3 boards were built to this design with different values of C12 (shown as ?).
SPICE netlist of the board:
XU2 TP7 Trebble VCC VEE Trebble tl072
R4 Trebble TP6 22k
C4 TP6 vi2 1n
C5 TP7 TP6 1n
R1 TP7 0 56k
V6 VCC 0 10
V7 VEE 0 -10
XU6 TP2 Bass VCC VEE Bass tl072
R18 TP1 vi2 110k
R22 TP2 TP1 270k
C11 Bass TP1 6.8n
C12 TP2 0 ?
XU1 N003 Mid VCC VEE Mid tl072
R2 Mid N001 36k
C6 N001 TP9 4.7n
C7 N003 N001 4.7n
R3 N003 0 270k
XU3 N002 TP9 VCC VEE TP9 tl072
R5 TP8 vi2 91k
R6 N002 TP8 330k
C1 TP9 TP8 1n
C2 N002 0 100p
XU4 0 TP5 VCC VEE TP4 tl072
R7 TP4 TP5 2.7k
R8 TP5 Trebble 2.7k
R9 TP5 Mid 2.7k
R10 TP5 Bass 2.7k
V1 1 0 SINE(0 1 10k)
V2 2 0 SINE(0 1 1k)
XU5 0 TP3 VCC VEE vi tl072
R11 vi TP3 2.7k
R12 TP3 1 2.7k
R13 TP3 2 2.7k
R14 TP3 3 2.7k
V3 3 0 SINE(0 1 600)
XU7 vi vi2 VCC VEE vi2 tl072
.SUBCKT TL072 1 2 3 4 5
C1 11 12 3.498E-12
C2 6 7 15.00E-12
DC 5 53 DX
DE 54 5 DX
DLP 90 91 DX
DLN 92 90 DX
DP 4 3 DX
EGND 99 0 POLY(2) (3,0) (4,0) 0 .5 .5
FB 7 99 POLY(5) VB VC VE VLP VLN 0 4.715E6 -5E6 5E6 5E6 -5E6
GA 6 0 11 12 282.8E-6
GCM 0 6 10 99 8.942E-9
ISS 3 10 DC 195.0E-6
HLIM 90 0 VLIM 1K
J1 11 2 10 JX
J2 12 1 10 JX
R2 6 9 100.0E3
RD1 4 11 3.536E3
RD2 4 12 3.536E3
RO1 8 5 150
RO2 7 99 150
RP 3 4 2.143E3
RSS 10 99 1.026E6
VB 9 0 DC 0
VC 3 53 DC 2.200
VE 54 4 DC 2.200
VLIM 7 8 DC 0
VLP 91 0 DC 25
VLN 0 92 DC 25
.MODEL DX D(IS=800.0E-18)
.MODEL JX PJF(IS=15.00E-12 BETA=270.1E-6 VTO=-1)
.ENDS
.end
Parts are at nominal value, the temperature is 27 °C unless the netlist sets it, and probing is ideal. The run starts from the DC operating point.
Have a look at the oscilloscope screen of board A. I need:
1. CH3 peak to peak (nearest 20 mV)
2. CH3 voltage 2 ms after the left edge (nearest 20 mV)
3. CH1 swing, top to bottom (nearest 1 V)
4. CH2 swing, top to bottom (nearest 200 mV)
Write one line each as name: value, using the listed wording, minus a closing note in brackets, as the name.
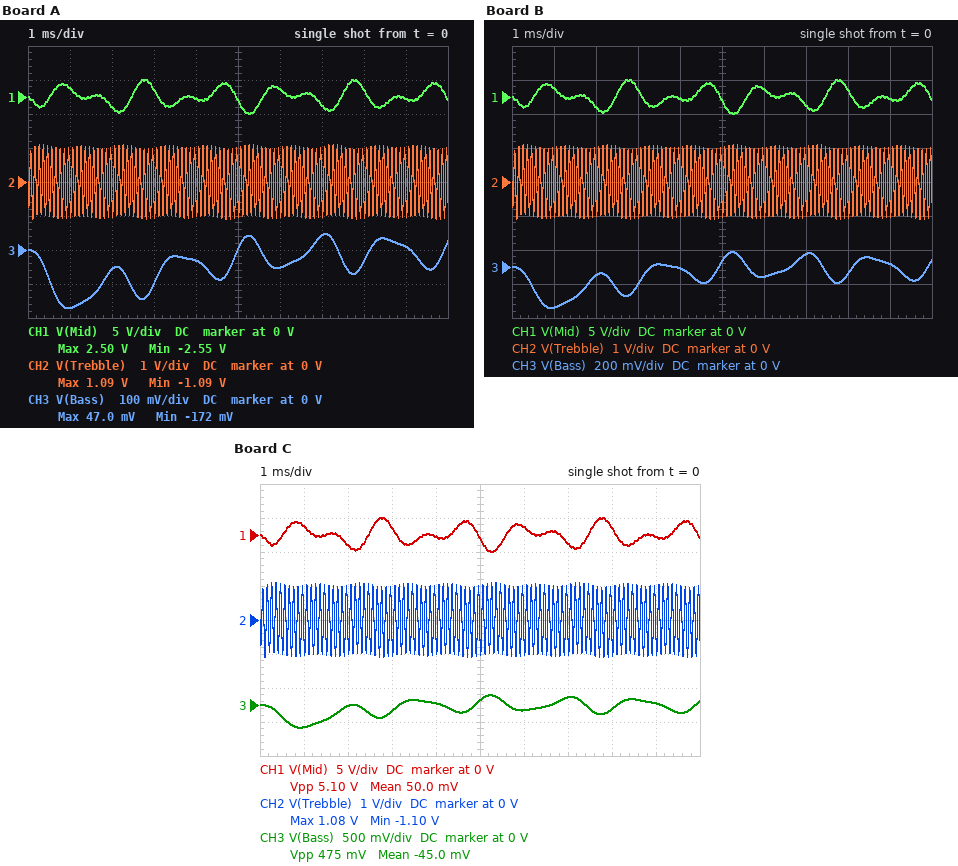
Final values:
CH3 peak to peak: 220 mV
CH3 voltage 2 ms after the left edge: -60 mV
CH1 swing, top to bottom: 5 V
CH2 swing, top to bottom: 2.2 V
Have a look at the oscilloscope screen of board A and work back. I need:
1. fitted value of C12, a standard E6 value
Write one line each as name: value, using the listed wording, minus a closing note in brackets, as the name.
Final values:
fitted value of C12, a standard E6 value: 6.8 nF
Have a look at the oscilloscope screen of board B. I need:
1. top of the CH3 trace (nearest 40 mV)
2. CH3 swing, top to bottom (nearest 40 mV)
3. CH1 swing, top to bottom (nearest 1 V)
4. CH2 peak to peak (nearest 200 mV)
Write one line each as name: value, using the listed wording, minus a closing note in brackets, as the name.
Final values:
top of the CH3 trace: 80 mV
CH3 swing, top to bottom: 320 mV
CH1 swing, top to bottom: 5 V
CH2 peak to peak: 2.2 V
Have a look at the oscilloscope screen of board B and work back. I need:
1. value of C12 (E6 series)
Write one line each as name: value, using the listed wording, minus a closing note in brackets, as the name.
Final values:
value of C12: 4.7 nF
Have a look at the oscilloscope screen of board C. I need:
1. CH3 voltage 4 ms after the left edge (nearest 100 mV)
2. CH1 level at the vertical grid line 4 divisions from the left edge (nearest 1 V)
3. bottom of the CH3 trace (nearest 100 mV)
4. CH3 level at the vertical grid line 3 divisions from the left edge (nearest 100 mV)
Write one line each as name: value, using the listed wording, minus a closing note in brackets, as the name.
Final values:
CH3 voltage 4 ms after the left edge: 0 V
CH1 level at the vertical grid line 4 divisions from the left edge: 0 V
bottom of the CH3 trace: -300 mV
CH3 level at the vertical grid line 3 divisions from the left edge: -100 mV
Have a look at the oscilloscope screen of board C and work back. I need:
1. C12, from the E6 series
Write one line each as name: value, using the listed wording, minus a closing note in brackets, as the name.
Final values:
C12, from the E6 series: 3.3 nF
